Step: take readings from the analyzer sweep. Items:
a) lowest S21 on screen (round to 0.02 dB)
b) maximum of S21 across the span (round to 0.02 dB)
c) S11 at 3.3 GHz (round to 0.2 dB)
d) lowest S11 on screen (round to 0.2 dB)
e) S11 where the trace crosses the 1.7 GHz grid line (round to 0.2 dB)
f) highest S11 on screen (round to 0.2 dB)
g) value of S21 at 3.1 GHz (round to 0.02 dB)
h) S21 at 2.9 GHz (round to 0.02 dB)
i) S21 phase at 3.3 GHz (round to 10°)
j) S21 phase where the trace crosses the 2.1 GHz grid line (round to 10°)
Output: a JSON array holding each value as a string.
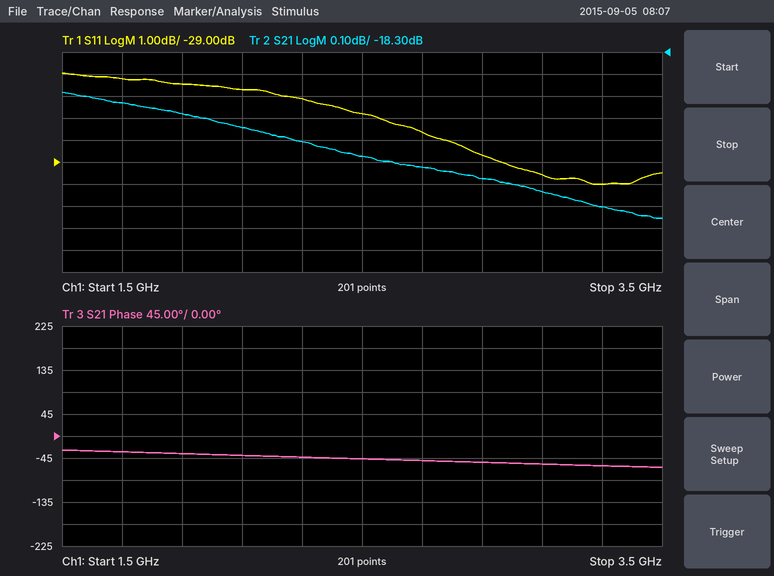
["-19.06 dB", "-18.48 dB", "-30.0 dB", "-30.0 dB", "-25.2 dB", "-25.0 dB", "-18.94 dB", "-18.88 dB", "-60°", "-40°"]
